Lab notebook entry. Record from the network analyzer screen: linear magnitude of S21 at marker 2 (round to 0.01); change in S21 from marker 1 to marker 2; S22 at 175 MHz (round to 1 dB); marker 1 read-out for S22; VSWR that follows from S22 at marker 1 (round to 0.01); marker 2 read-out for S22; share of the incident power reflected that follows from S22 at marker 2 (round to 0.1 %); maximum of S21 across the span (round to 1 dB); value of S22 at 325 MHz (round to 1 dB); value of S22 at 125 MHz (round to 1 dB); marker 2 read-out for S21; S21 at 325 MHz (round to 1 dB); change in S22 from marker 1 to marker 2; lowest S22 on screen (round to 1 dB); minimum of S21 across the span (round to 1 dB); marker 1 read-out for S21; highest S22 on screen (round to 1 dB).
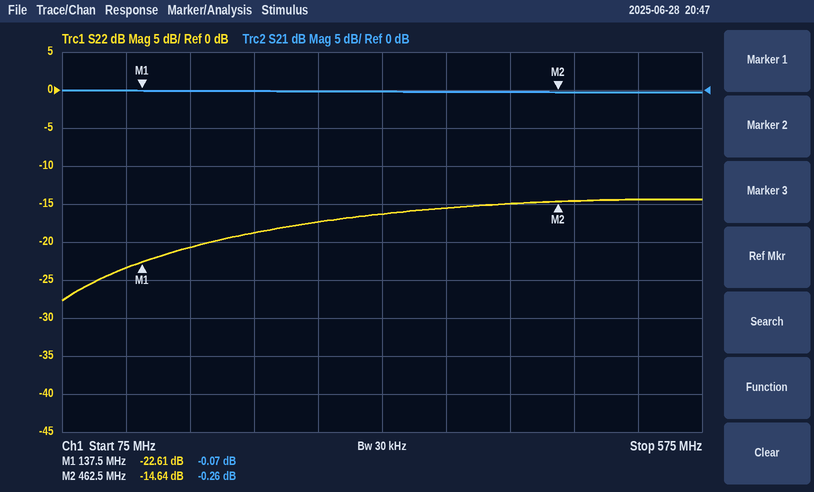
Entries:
0.97
-0.19 dB
-21 dB
-22.61 dB
1.16
-14.64 dB
3.4 %
0 dB
-16 dB
-23 dB
-0.26 dB
0 dB
7.97 dB
-28 dB
0 dB
-0.07 dB
-14 dB
